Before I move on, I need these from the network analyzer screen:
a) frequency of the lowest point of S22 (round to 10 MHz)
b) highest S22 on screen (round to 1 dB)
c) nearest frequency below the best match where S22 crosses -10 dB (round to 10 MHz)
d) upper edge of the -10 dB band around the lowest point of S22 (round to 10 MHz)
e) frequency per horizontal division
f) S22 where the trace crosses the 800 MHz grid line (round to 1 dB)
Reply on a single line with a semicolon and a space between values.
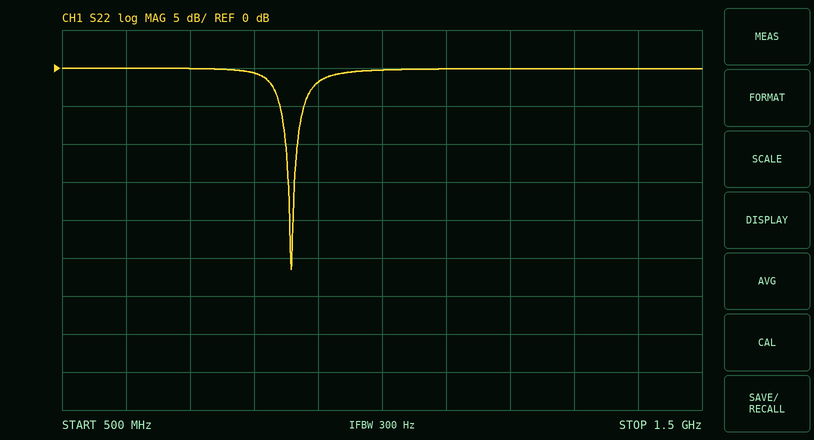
860 MHz; 0 dB; 850 MHz; 870 MHz; 100 MHz; -1 dB
